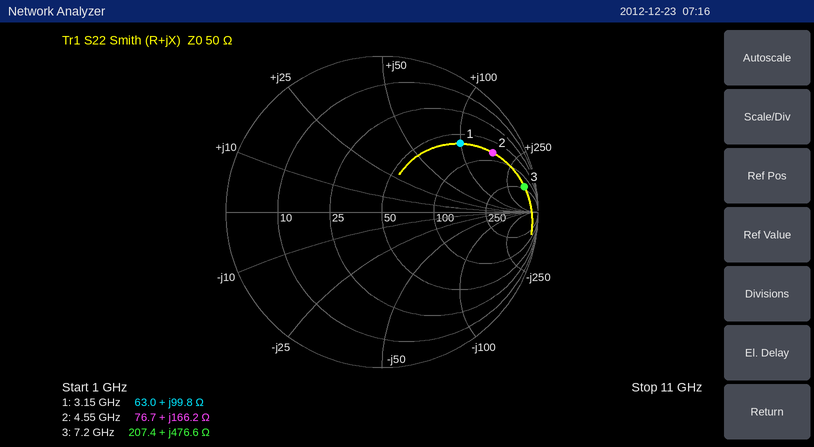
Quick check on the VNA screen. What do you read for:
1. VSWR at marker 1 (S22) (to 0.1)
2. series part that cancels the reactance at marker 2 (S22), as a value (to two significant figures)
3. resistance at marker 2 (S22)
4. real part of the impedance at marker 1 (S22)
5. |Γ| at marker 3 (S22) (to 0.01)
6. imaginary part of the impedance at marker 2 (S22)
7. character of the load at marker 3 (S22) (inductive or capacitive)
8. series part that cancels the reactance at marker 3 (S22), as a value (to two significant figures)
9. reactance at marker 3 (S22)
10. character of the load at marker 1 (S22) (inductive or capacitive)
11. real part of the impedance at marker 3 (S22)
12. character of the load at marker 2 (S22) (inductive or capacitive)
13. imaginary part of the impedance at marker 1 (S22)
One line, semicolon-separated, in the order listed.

5.0; 210 fF; 76.7 Ω; 63.0 Ω; 0.93; +166.2 Ω; inductive; 46 fF; +476.6 Ω; inductive; 207.4 Ω; inductive; +99.8 Ω
